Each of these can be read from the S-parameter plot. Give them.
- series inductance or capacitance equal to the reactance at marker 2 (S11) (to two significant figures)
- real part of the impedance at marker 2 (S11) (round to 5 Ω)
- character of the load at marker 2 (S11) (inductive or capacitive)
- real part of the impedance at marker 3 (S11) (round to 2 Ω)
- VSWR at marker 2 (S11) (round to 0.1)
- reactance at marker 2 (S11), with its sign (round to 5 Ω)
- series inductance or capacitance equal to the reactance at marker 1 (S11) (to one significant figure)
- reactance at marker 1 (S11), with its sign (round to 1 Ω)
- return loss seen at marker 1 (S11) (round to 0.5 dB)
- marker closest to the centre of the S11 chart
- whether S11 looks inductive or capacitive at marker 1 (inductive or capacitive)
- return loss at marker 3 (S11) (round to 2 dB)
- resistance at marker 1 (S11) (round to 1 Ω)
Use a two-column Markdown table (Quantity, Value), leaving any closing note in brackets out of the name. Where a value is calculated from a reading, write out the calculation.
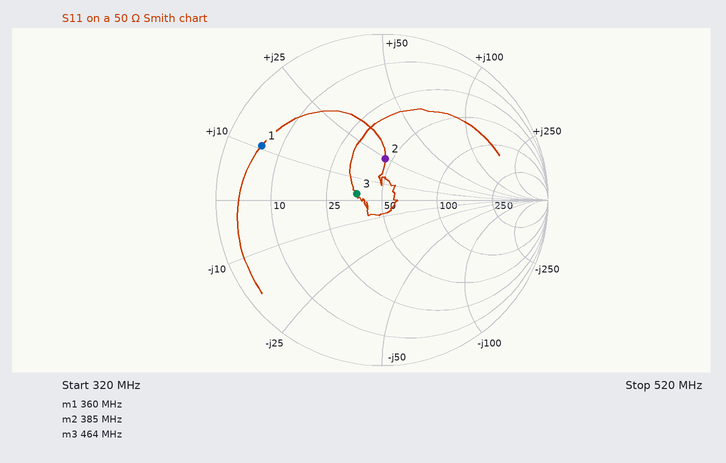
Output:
| Quantity | Value |
|---|---|
| series inductance or capacitance equal to the reactance at marker 2 (S11) | L = 25 Ω/(2π × 385 MHz) ≈ 10 nH |
| real part of the impedance at marker 2 (S11) | 45 Ω |
| character of the load at marker 2 (S11) | inductive |
| real part of the impedance at marker 3 (S11) | 36 Ω |
| VSWR at marker 2 (S11) | 1.7 |
| reactance at marker 2 (S11), with its sign | +25 Ω |
| series inductance or capacitance equal to the reactance at marker 1 (S11) | L = 11 Ω/(2π × 360 MHz) ≈ 5 nH |
| reactance at marker 1 (S11), with its sign | +11 Ω |
| return loss seen at marker 1 (S11) | 2.0 dB |
| marker closest to the centre of the S11 chart | marker 3 |
| whether S11 looks inductive or capacitive at marker 1 | inductive |
| return loss at marker 3 (S11) | 16 dB |
| resistance at marker 1 (S11) | 6 Ω |
